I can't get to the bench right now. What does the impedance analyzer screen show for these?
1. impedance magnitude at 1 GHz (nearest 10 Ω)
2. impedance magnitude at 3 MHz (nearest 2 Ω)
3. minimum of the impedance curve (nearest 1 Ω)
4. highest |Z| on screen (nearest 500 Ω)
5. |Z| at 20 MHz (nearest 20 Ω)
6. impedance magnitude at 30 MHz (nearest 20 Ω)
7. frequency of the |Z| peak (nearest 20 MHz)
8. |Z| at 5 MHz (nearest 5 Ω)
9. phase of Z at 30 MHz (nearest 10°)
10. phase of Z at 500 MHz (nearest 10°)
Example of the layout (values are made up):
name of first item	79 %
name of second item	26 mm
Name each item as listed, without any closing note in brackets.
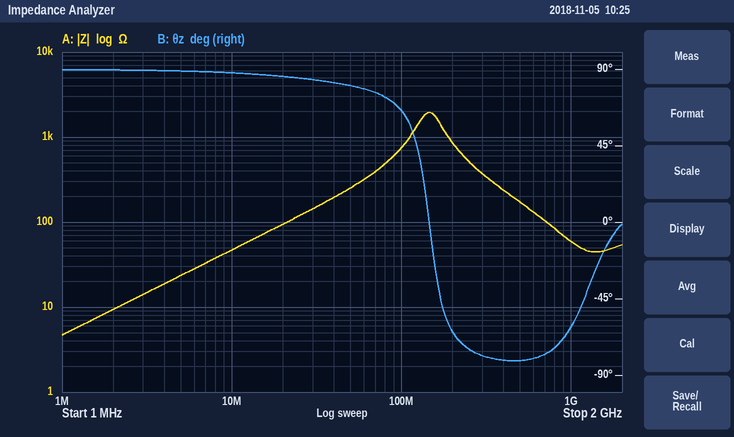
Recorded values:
impedance magnitude at 1 GHz	60 Ω
impedance magnitude at 3 MHz	14 Ω
minimum of the impedance curve	5 Ω
highest |Z| on screen	2.0 kΩ
|Z| at 20 MHz	100 Ω
impedance magnitude at 30 MHz	140 Ω
frequency of the |Z| peak	140 MHz
|Z| at 5 MHz	25 Ω
phase of Z at 30 MHz	80°
phase of Z at 500 MHz	-80°
